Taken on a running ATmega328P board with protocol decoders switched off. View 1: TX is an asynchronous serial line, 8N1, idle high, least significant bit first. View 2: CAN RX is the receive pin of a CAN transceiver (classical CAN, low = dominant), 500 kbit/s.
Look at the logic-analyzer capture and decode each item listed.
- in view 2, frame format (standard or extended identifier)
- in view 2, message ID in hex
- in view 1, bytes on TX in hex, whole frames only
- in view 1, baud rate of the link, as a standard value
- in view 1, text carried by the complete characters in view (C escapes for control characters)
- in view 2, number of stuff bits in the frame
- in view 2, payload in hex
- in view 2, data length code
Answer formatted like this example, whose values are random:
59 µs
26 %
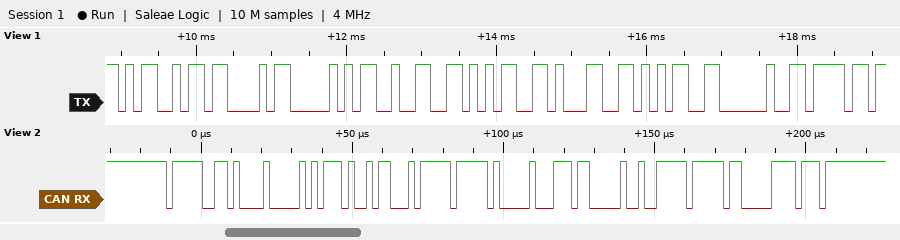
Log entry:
standard
0x7DA
0x4D 0x43 0x50 0x32 0x35 0x31 0x35 0x20 0x6F
9600 baud
"MCP2515 o"
9
17 4B 17 FF 00 EC 04 FF
8
